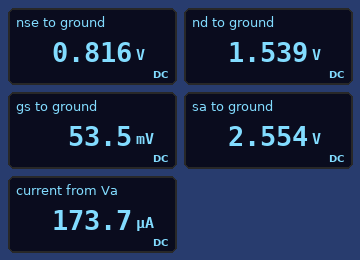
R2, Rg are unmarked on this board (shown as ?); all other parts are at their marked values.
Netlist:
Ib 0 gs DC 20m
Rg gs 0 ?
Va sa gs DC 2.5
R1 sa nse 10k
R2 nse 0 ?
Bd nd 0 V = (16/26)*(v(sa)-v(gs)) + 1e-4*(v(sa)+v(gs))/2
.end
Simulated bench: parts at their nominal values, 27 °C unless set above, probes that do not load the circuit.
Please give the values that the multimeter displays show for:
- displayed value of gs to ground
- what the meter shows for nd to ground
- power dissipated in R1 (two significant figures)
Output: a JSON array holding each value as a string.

["53.5 mV", "1.539 V", "300 µW"]
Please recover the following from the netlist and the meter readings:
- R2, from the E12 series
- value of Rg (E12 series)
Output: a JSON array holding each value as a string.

["4.7 kΩ", "2.7 Ω"]
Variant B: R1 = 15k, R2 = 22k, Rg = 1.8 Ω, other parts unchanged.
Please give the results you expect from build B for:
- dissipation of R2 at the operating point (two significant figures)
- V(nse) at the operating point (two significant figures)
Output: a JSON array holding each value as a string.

["100 µW", "1.5 V"]
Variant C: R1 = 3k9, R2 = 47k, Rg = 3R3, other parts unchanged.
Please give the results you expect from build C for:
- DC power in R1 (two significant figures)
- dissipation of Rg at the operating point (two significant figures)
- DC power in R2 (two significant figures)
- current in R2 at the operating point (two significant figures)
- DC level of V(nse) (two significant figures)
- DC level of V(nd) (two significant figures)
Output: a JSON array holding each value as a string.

["9.9 µW", "1.3 mW", "120 µW", "50 µA", "2.4 V", "1.5 V"]
